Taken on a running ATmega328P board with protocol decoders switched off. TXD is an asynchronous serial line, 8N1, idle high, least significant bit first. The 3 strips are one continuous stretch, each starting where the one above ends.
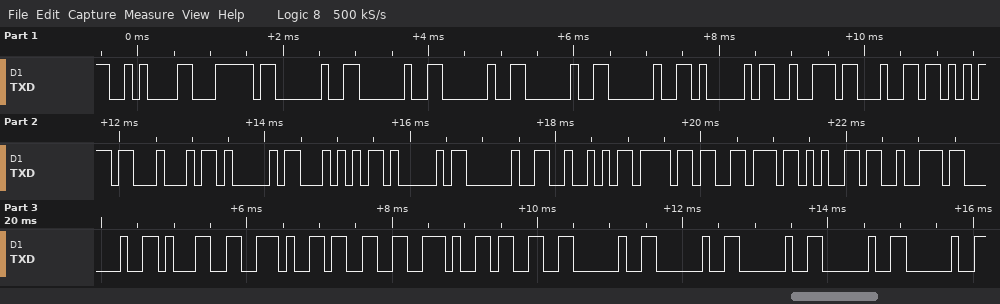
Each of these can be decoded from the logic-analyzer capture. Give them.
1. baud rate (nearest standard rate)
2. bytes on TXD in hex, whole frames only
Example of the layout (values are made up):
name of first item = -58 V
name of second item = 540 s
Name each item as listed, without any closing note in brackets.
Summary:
baud rate = 9600 baud
bytes on TXD in hex, whole frames only = 0A 7C 20 20 20 20 20 41 72 64 75 44 41 54 41 20 52 6F 76 65 72 20 31 2E 33 2E 33 20 20 20 20 20
